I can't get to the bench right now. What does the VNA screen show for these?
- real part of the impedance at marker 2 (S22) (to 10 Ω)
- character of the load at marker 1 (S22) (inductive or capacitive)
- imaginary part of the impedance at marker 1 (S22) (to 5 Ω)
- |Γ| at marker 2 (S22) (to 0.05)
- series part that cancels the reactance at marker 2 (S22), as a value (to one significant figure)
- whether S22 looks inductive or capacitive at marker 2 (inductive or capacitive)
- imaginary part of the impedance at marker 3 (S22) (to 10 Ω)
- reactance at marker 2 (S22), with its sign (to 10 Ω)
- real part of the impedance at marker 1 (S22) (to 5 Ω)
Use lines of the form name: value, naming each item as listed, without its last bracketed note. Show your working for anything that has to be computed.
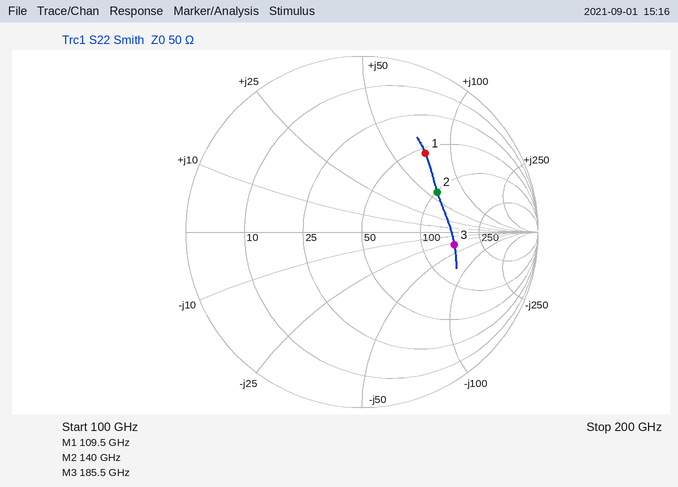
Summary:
real part of the impedance at marker 2 (S22): 100 Ω
character of the load at marker 1 (S22): inductive
imaginary part of the impedance at marker 1 (S22): +75 Ω
|Γ| at marker 2 (S22): 0.50
series part that cancels the reactance at marker 2 (S22), as a value: C = 1/(2π × 140 GHz × 60 Ω) ≈ 18.9 fF, so 20 fF to one significant figure
whether S22 looks inductive or capacitive at marker 2: inductive
imaginary part of the impedance at marker 3 (S22): -30 Ω
reactance at marker 2 (S22), with its sign: +60 Ω
real part of the impedance at marker 1 (S22): 55 Ω
